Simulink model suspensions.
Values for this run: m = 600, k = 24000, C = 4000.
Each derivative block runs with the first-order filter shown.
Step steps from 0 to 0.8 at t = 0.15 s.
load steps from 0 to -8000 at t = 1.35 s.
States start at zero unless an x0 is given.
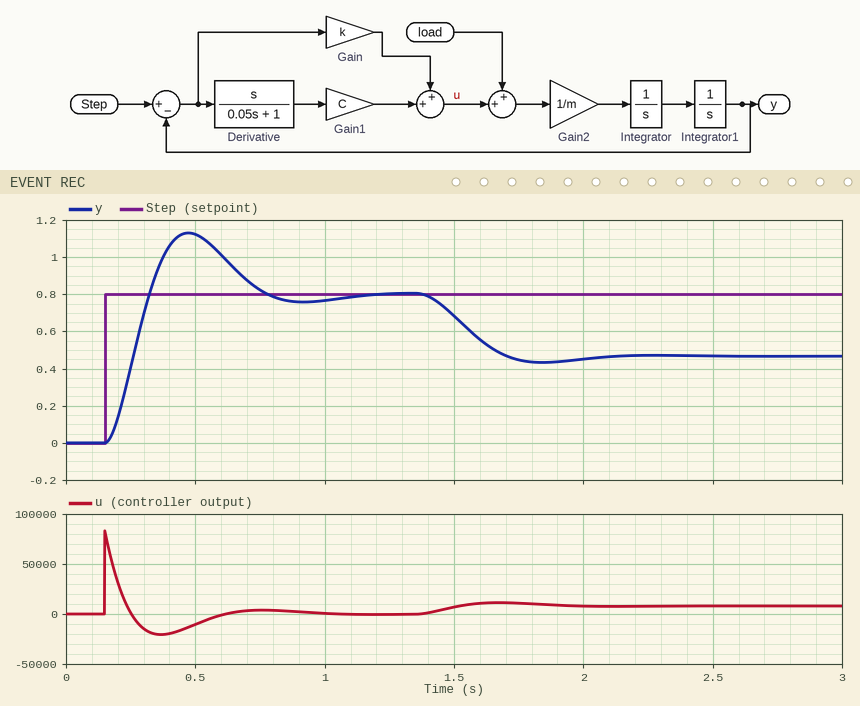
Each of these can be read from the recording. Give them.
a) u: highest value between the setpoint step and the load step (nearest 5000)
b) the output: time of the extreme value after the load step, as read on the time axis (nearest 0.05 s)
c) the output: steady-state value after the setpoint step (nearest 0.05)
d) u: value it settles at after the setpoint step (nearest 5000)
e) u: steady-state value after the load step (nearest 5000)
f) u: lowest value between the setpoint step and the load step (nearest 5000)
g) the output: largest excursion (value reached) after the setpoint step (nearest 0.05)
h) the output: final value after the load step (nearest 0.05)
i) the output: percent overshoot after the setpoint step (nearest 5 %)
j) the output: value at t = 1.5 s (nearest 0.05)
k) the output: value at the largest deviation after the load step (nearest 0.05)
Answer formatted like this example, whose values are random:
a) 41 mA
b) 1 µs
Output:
a) 85000
b) 1.85 s
c) 0.80
d) 0
e) 10000
f) -20000
g) 1.15
h) 0.45
i) 40 %
j) 0.70
k) 0.45
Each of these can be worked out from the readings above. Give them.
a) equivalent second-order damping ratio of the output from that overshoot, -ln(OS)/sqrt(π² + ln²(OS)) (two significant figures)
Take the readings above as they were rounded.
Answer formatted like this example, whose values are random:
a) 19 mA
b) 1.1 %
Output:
a) 0.28
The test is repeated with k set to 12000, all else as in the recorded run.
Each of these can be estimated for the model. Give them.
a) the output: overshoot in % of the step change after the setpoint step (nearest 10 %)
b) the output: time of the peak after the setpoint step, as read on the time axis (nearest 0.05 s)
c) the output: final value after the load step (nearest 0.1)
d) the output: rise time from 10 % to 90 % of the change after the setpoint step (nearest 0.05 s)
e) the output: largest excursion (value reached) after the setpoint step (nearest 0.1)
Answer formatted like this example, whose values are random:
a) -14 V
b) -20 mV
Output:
a) 30 %
b) 0.55 s
c) 0.1
d) 0.15 s
e) 1.0
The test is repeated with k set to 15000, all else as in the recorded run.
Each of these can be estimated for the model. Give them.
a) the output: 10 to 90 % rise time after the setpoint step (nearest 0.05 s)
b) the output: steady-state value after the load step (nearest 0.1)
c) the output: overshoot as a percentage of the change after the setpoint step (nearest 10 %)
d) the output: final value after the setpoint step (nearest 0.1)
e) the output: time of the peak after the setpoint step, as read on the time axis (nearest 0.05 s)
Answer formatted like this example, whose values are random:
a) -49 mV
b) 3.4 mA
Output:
a) 0.15 s
b) 0.3
c) 30 %
d) 0.8
e) 0.50 s
